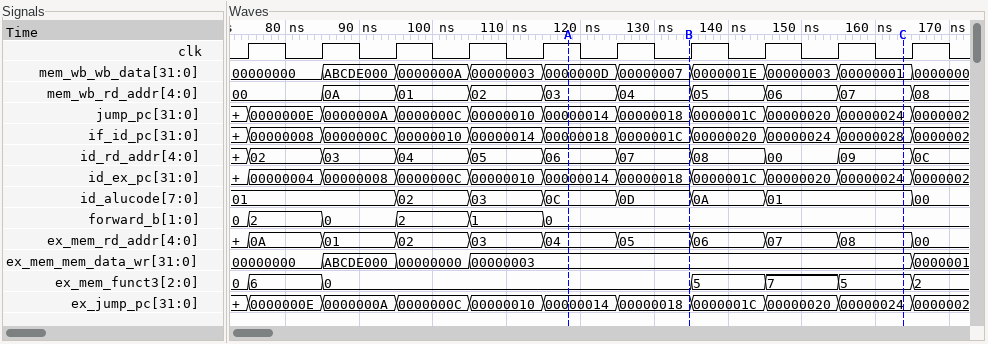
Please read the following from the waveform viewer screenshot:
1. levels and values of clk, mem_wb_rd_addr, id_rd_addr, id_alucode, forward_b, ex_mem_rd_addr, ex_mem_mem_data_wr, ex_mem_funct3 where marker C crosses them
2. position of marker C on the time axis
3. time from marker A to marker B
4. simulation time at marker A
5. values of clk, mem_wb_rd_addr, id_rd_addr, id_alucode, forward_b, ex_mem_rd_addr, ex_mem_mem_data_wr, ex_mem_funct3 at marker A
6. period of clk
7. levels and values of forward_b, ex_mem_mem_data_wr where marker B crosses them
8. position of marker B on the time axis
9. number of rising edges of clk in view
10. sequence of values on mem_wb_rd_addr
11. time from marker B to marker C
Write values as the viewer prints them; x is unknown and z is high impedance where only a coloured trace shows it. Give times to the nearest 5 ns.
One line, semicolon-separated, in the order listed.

clk=0, mem_wb_rd_addr=07, id_rd_addr=09, id_alucode=01, forward_b=0, ex_mem_rd_addr=08, ex_mem_mem_data_wr=00000003, ex_mem_funct3=5; 165 ns; 15 ns; 120 ns; clk=1, mem_wb_rd_addr=03, id_rd_addr=06, id_alucode=0C, forward_b=0, ex_mem_rd_addr=04, ex_mem_mem_data_wr=00000003, ex_mem_funct3=0; 10 ns; forward_b=0, ex_mem_mem_data_wr=00000003; 135 ns; 10; 00, 0A, 01, 02, 03, 04, 05, 06, 07, 08; 30 ns
